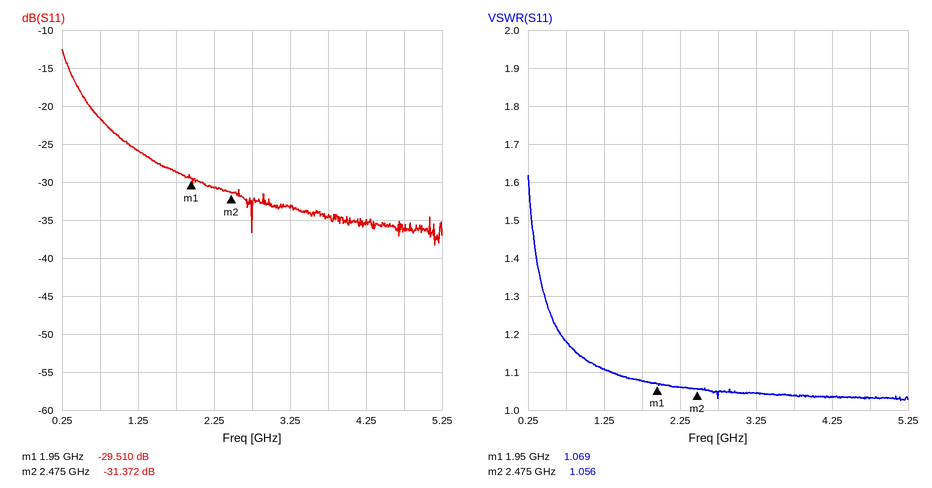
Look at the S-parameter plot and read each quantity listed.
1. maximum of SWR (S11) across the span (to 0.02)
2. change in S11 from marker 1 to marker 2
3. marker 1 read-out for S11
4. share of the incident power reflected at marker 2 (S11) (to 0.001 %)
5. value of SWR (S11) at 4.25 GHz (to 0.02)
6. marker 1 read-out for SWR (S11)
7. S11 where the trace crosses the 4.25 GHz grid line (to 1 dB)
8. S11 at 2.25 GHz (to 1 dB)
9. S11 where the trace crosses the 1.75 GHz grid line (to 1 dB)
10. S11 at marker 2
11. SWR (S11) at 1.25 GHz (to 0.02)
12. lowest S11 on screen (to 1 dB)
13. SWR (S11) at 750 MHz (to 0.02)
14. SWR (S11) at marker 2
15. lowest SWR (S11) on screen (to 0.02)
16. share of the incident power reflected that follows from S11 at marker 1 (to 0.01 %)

1.62
-1.862 dB
-29.510 dB
0.073 %
1.04
1.069
-35 dB
-31 dB
-29 dB
-31.372 dB
1.10
-38 dB
1.18
1.056
1.02
0.11 %
